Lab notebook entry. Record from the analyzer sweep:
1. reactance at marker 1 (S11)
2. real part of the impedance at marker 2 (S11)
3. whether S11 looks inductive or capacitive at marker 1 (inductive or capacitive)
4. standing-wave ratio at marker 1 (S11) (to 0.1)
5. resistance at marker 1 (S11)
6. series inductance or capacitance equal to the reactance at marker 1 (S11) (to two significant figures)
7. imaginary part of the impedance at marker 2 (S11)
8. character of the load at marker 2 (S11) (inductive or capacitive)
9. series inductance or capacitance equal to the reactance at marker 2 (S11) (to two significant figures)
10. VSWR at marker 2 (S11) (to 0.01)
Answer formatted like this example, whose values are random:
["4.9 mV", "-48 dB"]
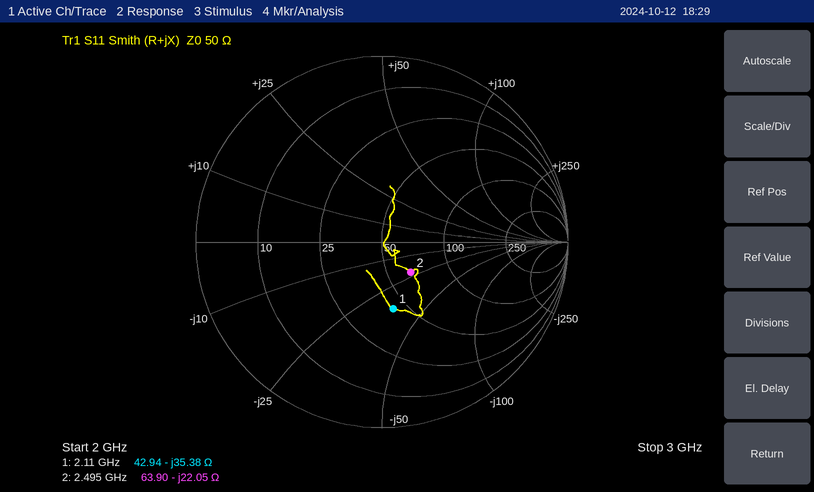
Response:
["-35.38 Ω", "63.90 Ω", "capacitive", "2.1", "42.94 Ω", "2.1 pF", "-22.05 Ω", "capacitive", "2.9 pF", "1.58"]
